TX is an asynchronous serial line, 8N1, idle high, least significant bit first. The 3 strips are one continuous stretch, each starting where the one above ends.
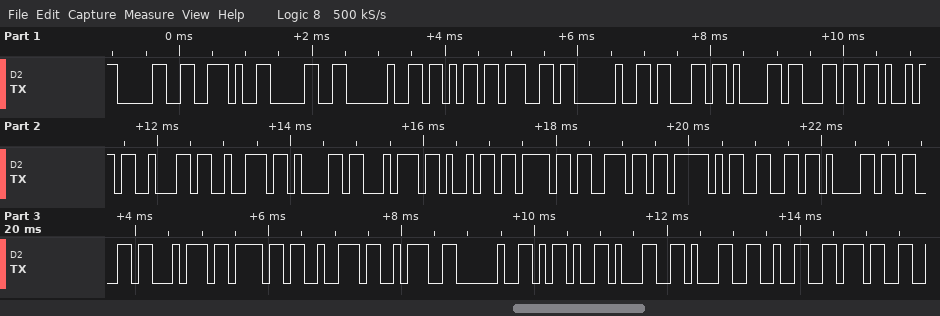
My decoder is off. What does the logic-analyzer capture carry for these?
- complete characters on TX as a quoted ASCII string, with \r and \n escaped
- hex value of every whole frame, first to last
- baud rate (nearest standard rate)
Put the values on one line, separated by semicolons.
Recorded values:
"0.0 kg calibration_factor: -1127"; 30 2E 30 20 6B 67 20 63 61 6C 69 62 72 61 74 69 6F 6E 5F 66 61 63 74 6F 72 3A 20 2D 31 31 32 37; 9600 baud
